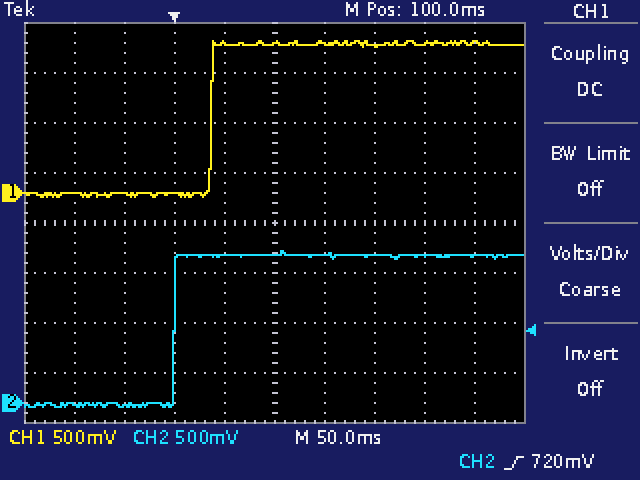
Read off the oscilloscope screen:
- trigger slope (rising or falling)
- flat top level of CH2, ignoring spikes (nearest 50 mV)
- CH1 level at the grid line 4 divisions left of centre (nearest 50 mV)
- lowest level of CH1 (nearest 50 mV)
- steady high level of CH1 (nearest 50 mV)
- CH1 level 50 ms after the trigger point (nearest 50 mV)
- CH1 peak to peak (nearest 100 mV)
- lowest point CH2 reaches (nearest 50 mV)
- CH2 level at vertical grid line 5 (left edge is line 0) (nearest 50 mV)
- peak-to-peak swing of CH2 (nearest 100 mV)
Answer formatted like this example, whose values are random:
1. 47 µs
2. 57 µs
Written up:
1. rising
2. 1.50 V
3. 0 mV
4. -50 mV
5. 1.50 V
6. 1.50 V
7. 1.60 V
8. -50 mV
9. 1.50 V
10. 1.60 V
